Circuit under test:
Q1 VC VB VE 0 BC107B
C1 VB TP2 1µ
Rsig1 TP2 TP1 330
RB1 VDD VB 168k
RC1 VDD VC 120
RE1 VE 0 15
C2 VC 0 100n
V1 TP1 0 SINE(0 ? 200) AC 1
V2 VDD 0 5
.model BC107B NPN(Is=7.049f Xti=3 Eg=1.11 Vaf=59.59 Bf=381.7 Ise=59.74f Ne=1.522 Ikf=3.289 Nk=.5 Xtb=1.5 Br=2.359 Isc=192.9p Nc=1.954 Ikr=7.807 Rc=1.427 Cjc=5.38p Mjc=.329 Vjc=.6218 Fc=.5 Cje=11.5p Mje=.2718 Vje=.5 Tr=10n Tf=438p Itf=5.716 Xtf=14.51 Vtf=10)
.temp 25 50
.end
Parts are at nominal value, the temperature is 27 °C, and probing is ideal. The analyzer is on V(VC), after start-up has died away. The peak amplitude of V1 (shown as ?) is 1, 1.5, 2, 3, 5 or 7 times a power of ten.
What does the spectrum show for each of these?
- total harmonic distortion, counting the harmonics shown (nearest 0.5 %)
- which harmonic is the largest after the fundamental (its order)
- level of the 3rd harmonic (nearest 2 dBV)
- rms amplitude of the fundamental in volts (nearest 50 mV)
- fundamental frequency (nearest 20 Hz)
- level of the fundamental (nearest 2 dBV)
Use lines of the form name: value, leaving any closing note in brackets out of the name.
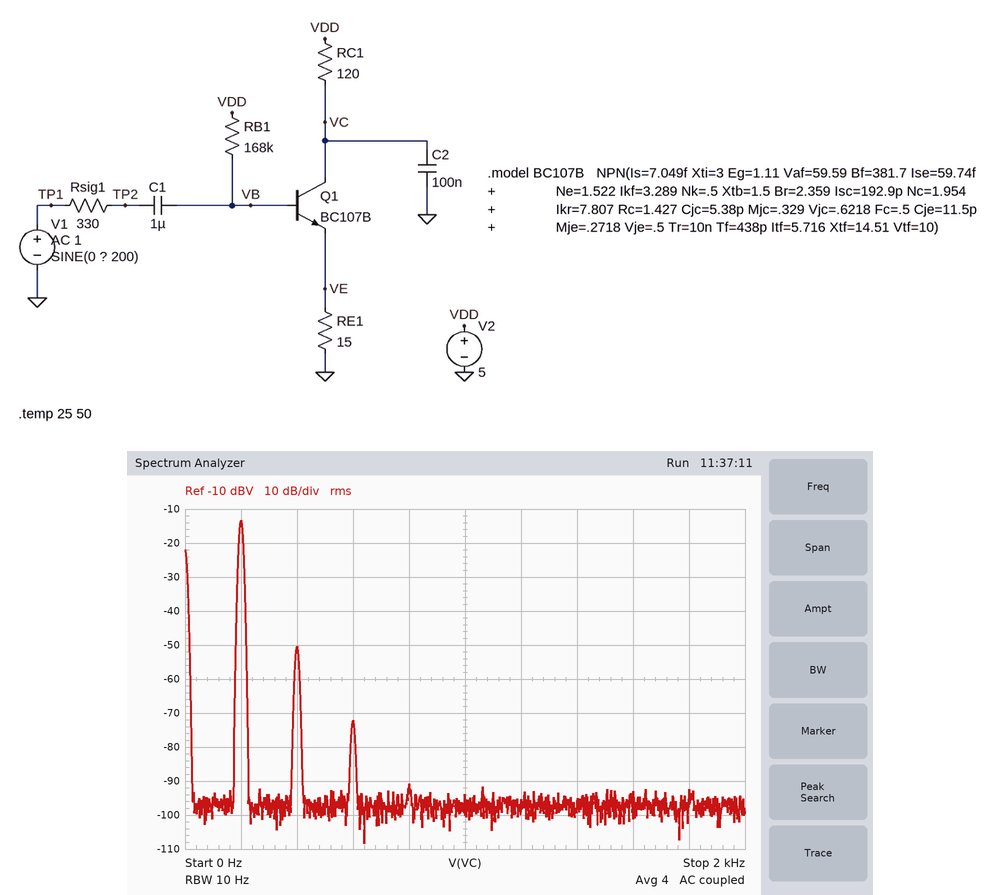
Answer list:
total harmonic distortion, counting the harmonics shown: 1.5 %
which harmonic is the largest after the fundamental: 2
level of the 3rd harmonic: -72 dBV
rms amplitude of the fundamental in volts: 200 mV
fundamental frequency: 200 Hz
level of the fundamental: -14 dBV
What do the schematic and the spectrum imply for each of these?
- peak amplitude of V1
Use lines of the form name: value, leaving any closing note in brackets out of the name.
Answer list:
peak amplitude of V1: 50 mV
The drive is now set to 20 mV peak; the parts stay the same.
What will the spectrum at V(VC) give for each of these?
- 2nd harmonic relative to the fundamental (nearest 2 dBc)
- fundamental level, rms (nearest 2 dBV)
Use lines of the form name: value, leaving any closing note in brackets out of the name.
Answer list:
2nd harmonic relative to the fundamental: -46 dBc
fundamental level, rms: -22 dBV
